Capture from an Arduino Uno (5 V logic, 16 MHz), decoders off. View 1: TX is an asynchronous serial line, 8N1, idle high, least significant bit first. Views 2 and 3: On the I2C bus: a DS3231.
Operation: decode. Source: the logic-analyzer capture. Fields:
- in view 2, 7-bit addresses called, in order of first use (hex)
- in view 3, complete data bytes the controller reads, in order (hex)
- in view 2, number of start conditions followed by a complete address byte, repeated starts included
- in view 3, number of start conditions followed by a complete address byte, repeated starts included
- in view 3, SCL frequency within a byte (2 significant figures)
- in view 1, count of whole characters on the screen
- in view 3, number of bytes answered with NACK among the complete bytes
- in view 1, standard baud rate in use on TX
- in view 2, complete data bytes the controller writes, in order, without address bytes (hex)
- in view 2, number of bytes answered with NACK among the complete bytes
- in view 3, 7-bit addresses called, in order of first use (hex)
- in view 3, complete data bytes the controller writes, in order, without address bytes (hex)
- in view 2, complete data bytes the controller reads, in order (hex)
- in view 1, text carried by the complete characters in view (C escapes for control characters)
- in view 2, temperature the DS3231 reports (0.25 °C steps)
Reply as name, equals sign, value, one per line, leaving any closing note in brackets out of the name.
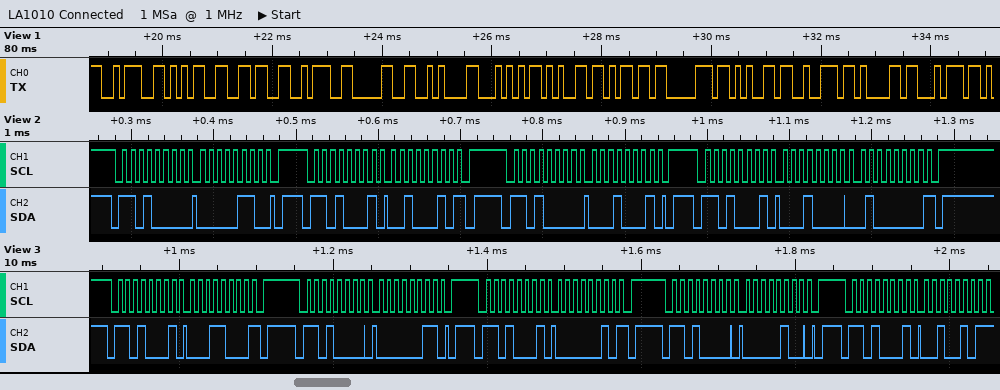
in view 2, 7-bit addresses called, in order of first use = 0x68
in view 3, complete data bytes the controller reads, in order = 18 02 25
in view 2, number of start conditions followed by a complete address byte, repeated starts included = 4
in view 3, number of start conditions followed by a complete address byte, repeated starts included = 5
in view 3, SCL frequency within a byte = 100 kHz
in view 1, count of whole characters on the screen = 14
in view 3, number of bytes answered with NACK among the complete bytes = 3
in view 1, standard baud rate in use on TX = 9600 baud
in view 2, complete data bytes the controller writes, in order, without address bytes = 06 11
in view 2, number of bytes answered with NACK among the complete bytes = 2
in view 3, 7-bit addresses called, in order of first use = 0x68
in view 3, complete data bytes the controller writes, in order, without address bytes = 03 04
in view 2, complete data bytes the controller reads, in order = 22 10 40
in view 1, text carried by the complete characters in view = ":56:0\nTemperat"
in view 2, temperature the DS3231 reports = 16.25 °C
